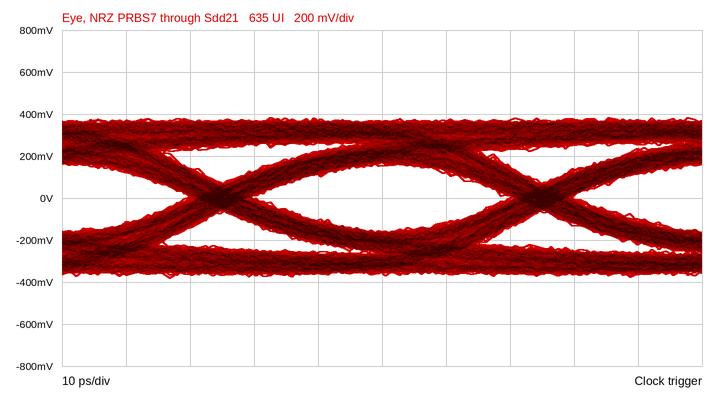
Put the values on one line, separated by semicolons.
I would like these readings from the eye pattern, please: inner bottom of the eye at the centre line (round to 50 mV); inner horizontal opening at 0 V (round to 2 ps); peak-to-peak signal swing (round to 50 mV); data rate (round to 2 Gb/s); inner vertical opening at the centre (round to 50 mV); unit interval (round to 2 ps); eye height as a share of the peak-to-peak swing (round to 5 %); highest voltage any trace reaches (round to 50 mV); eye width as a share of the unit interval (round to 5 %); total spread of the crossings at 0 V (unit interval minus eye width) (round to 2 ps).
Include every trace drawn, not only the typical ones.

-150 mV; 40 ps; 750 mV; 20 Gb/s; 300 mV; 50 ps; 40 %; 400 mV; 80 %; 10 ps
